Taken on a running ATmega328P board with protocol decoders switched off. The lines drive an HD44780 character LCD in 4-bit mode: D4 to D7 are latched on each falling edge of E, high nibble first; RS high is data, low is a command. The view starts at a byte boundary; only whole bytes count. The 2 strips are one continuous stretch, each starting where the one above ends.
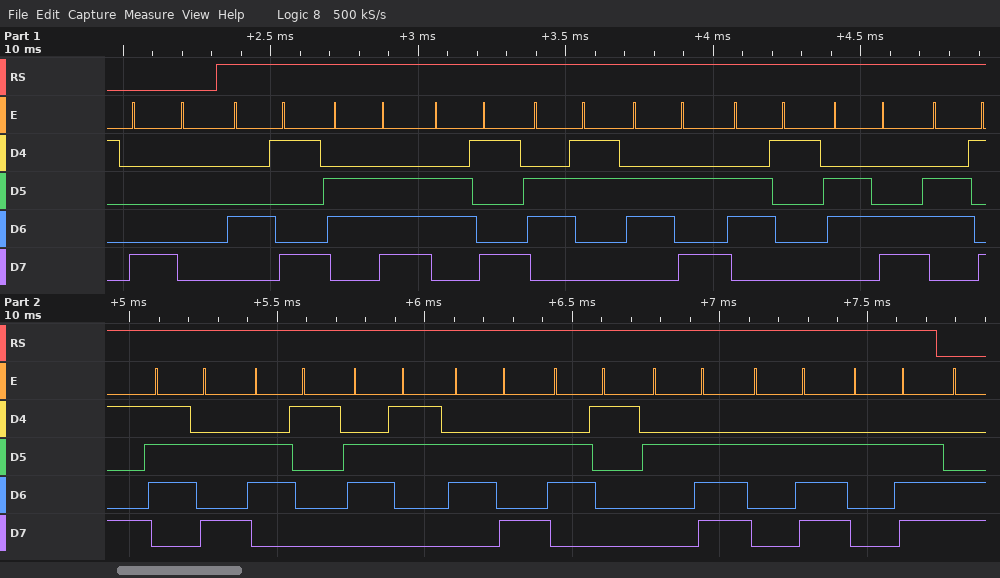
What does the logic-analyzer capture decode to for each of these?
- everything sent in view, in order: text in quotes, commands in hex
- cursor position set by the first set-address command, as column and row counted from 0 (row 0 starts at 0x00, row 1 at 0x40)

0x80 "Inicjalizacja..."
column 0, row 0
